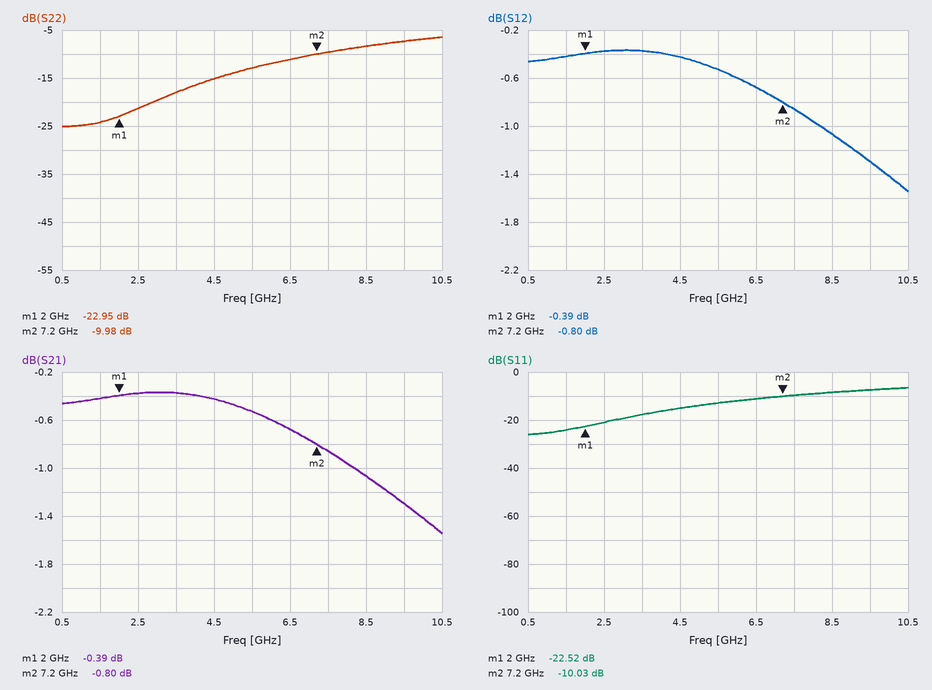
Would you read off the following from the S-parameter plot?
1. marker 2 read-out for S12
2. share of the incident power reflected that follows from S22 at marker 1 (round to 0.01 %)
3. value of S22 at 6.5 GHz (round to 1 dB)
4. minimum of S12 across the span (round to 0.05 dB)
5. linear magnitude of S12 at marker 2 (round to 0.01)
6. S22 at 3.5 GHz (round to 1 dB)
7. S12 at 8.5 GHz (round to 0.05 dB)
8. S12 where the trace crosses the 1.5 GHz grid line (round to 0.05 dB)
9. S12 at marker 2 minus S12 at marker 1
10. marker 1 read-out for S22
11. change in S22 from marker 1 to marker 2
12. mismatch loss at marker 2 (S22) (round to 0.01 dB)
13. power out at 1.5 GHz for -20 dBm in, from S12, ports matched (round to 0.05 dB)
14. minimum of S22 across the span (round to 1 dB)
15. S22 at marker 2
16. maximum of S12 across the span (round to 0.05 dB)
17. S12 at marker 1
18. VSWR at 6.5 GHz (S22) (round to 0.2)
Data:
-0.80 dB
0.51 %
-11 dB
-1.55 dB
0.91
-18 dB
-1.05 dB
-0.40 dB
-0.41 dB
-22.95 dB
12.97 dB
0.46 dB
-20.40 dBm
-25 dB
-9.98 dB
-0.35 dB
-0.39 dB
1.8
